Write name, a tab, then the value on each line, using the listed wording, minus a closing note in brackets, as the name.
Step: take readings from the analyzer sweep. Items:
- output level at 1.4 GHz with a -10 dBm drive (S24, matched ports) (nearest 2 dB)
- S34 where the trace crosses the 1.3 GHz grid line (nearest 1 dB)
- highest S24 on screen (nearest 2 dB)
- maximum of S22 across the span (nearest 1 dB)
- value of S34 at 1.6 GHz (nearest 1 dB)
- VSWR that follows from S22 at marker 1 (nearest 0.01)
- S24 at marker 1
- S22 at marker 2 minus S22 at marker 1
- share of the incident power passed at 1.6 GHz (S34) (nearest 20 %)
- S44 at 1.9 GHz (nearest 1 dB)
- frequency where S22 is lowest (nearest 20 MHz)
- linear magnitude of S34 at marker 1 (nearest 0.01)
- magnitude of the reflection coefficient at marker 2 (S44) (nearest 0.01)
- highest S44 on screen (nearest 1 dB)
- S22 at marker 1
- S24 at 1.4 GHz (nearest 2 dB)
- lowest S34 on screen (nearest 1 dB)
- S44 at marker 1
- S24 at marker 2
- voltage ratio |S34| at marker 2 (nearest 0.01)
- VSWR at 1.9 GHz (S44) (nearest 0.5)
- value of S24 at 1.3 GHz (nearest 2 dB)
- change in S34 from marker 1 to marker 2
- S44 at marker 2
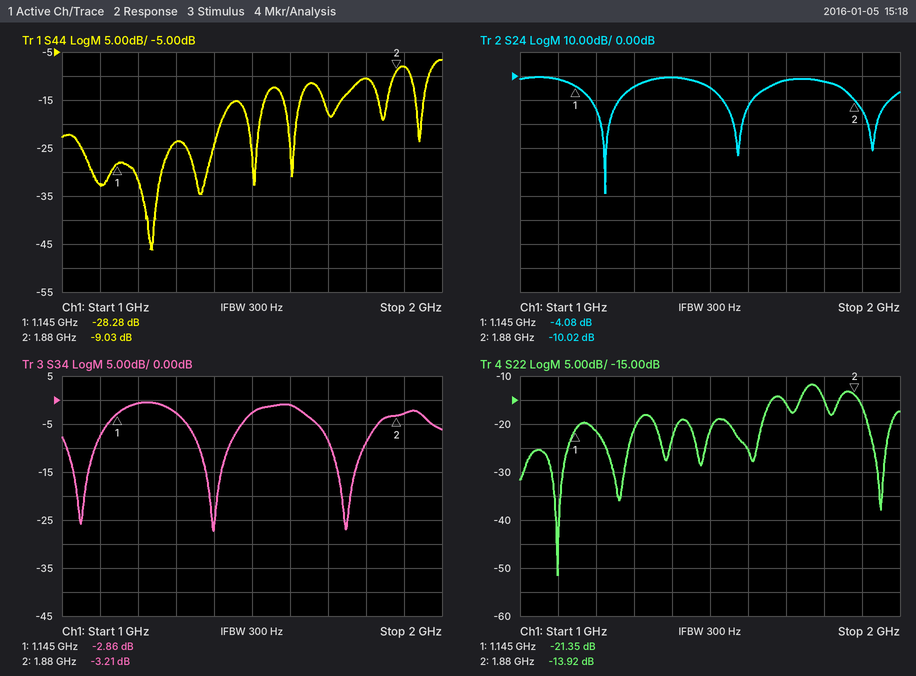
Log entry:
output level at 1.4 GHz with a -10 dBm drive (S24, matched ports)	-10 dBm
S34 where the trace crosses the 1.3 GHz grid line	-3 dB
highest S24 on screen	0 dB
maximum of S22 across the span	-12 dB
value of S34 at 1.6 GHz	-1 dB
VSWR that follows from S22 at marker 1	1.19
S24 at marker 1	-4.08 dB
S22 at marker 2 minus S22 at marker 1	7.43 dB
share of the incident power passed at 1.6 GHz (S34)	80 %
S44 at 1.9 GHz	-8 dB
frequency where S22 is lowest	1.10 GHz
linear magnitude of S34 at marker 1	0.72
magnitude of the reflection coefficient at marker 2 (S44)	0.35
highest S44 on screen	-7 dB
S22 at marker 1	-21.35 dB
S24 at 1.4 GHz	0 dB
lowest S34 on screen	-27 dB
S44 at marker 1	-28.28 dB
S24 at marker 2	-10.02 dB
voltage ratio |S34| at marker 2	0.69
VSWR at 1.9 GHz (S44)	2.5
value of S24 at 1.3 GHz	-4 dB
change in S34 from marker 1 to marker 2	-0.35 dB
S44 at marker 2	-9.03 dB
